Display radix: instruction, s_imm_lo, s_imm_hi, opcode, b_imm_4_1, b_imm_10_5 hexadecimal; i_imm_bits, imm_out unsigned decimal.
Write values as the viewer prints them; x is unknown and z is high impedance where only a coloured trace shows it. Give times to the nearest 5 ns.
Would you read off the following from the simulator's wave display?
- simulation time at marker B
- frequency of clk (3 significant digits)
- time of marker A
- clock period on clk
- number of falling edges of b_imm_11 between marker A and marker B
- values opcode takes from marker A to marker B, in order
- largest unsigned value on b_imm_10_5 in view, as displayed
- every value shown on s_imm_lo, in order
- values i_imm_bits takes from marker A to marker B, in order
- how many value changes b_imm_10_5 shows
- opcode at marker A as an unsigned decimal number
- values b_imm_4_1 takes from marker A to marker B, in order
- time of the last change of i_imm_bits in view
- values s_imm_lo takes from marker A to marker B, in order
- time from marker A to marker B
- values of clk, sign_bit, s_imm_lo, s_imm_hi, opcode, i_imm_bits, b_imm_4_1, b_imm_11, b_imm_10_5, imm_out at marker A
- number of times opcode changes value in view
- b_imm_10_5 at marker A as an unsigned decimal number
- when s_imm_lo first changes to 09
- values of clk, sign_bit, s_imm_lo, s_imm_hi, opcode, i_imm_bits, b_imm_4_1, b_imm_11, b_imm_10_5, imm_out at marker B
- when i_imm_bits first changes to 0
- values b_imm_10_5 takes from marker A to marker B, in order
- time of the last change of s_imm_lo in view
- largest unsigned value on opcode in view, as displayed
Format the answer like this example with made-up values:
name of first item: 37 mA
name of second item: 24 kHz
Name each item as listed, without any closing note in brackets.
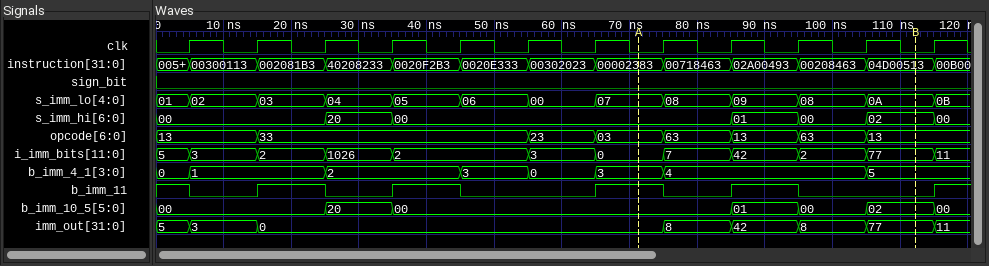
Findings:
simulation time at marker B: 110 ns
frequency of clk: 100 MHz
time of marker A: 70 ns
clock period on clk: 10 ns
number of falling edges of b_imm_11 between marker A and marker B: 2
values opcode takes from marker A to marker B, in order: 03, 63, 13, 63, 13
largest unsigned value on b_imm_10_5 in view, as displayed: 20
every value shown on s_imm_lo, in order: 01, 02, 03, 04, 05, 06, 00, 07, 08, 09, 08, 0A, 0B
values i_imm_bits takes from marker A to marker B, in order: 0, 7, 42, 2, 77
how many value changes b_imm_10_5 shows: 6
opcode at marker A as an unsigned decimal number: 3
values b_imm_4_1 takes from marker A to marker B, in order: 3, 4, 5
time of the last change of i_imm_bits in view: 115 ns
values s_imm_lo takes from marker A to marker B, in order: 07, 08, 09, 08, 0A
time from marker A to marker B: 40 ns
values of clk, sign_bit, s_imm_lo, s_imm_hi, opcode, i_imm_bits, b_imm_4_1, b_imm_11, b_imm_10_5, imm_out at marker A: clk=0, sign_bit=0, s_imm_lo=07, s_imm_hi=00, opcode=03, i_imm_bits=0, b_imm_4_1=3, b_imm_11=1, b_imm_10_5=00, imm_out=0
number of times opcode changes value in view: 7
b_imm_10_5 at marker A as an unsigned decimal number: 0
when s_imm_lo first changes to 09: 85 ns
values of clk, sign_bit, s_imm_lo, s_imm_hi, opcode, i_imm_bits, b_imm_4_1, b_imm_11, b_imm_10_5, imm_out at marker B: clk=0, sign_bit=0, s_imm_lo=0A, s_imm_hi=02, opcode=13, i_imm_bits=77, b_imm_4_1=5, b_imm_11=0, b_imm_10_5=02, imm_out=77
when i_imm_bits first changes to 0: 65 ns
values b_imm_10_5 takes from marker A to marker B, in order: 00, 01, 00, 02
time of the last change of s_imm_lo in view: 115 ns
largest unsigned value on opcode in view, as displayed: 63
